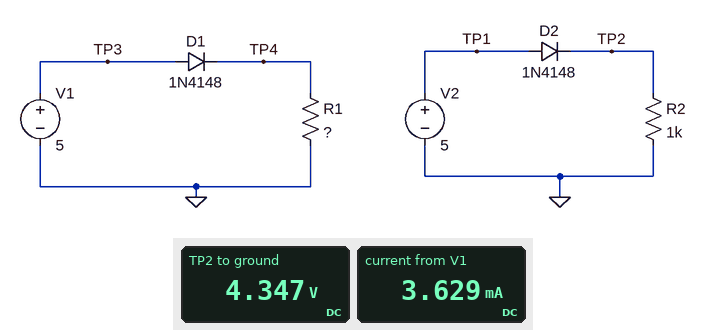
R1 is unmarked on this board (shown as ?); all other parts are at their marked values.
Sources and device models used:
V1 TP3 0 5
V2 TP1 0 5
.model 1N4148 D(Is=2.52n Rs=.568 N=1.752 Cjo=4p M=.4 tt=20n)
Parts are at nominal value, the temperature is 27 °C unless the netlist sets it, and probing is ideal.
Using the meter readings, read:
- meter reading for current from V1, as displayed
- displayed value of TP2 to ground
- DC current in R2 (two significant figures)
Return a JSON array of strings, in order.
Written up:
["3.629 mA", "4.347 V", "4.3 mA"]
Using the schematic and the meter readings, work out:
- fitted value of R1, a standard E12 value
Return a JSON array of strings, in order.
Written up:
["1.2 kΩ"]
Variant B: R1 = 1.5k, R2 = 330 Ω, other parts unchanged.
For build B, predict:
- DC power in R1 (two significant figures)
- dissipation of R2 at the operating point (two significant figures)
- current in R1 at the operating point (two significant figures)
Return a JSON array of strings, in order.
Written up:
["13 mW", "56 mW", "2.9 mA"]
